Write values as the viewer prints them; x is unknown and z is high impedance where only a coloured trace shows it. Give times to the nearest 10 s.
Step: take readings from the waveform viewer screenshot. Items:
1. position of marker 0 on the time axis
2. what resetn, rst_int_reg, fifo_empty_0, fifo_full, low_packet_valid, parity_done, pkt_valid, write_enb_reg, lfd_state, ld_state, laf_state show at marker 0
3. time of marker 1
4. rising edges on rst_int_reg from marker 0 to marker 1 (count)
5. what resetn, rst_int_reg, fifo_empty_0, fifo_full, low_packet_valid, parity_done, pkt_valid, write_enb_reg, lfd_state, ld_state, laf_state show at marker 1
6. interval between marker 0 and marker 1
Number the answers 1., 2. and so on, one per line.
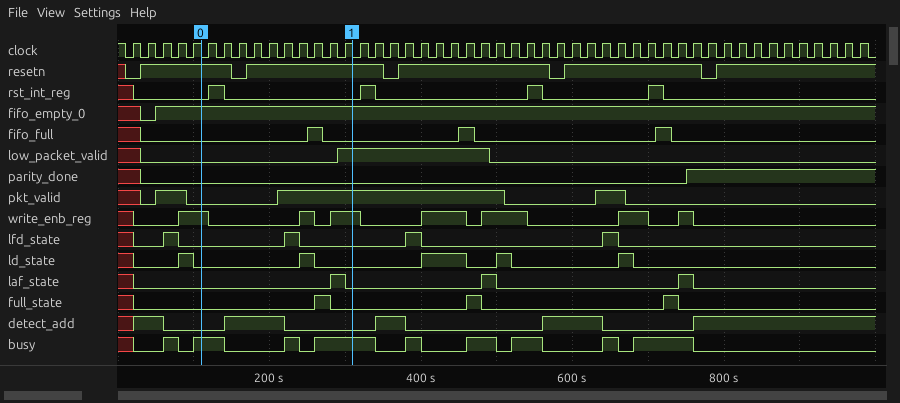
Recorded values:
1. 110 s
2. resetn=1, rst_int_reg=0, fifo_empty_0=1, fifo_full=0, low_packet_valid=0, parity_done=0, pkt_valid=0, write_enb_reg=1, lfd_state=0, ld_state=0, laf_state=0
3. 310 s
4. 1
5. resetn=1, rst_int_reg=0, fifo_empty_0=1, fifo_full=0, low_packet_valid=1, parity_done=0, pkt_valid=1, write_enb_reg=1, lfd_state=0, ld_state=0, laf_state=0
6. 200 s
